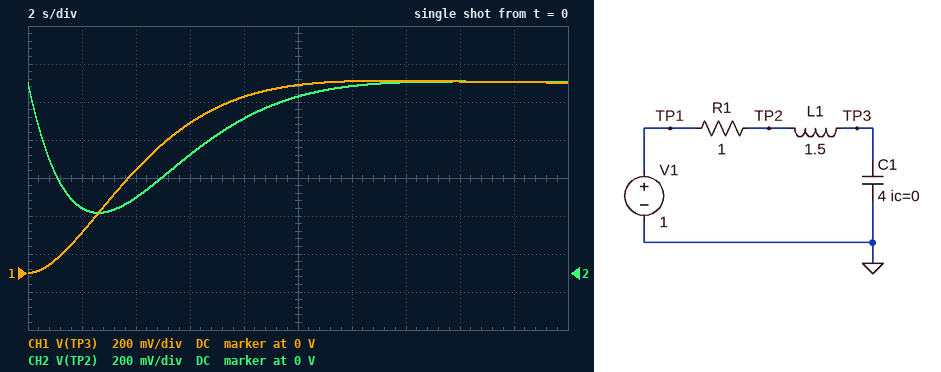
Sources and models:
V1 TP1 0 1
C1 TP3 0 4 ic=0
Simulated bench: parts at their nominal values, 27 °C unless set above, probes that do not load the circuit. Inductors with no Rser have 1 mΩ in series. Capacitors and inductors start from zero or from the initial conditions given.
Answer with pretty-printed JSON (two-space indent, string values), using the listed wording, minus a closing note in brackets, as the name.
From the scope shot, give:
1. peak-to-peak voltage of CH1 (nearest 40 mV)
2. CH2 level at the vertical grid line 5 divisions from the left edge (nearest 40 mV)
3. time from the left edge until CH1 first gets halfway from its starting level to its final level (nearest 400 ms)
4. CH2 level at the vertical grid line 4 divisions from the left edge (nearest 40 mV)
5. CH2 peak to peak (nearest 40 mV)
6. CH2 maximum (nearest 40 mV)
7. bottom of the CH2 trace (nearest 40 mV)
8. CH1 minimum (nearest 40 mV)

{
  "peak-to-peak voltage of CH1": "1.00 V",
  "CH2 level at the vertical grid line 5 divisions from the left edge": "920 mV",
  "time from the left edge until CH1 first gets halfway from its starting level to its final level": "3.6 s",
  "CH2 level at the vertical grid line 4 divisions from the left edge": "800 mV",
  "CH2 peak to peak": "680 mV",
  "CH2 maximum": "1.00 V",
  "bottom of the CH2 trace": "320 mV",
  "CH1 minimum": "0 V"
}
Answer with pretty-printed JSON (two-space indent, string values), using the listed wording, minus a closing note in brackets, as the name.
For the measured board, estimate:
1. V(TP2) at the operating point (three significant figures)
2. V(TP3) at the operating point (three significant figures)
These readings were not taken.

{
  "V(TP2) at the operating point": "1.00 V",
  "V(TP3) at the operating point": "1.00 V"
}
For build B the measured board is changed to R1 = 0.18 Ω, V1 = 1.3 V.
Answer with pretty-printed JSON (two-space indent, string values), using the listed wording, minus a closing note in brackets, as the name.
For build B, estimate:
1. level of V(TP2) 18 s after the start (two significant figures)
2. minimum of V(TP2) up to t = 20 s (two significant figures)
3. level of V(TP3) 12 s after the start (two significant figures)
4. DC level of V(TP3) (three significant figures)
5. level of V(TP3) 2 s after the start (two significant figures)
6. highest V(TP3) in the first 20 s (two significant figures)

{
  "level of V(TP2) 18 s after the start": "1.2 V",
  "minimum of V(TP2) up to t = 20 s": "990 mV",
  "level of V(TP3) 12 s after the start": "1.3 V",
  "DC level of V(TP3)": "1.30 V",
  "level of V(TP3) 2 s after the start": "380 mV",
  "highest V(TP3) in the first 20 s": "2.1 V"
}
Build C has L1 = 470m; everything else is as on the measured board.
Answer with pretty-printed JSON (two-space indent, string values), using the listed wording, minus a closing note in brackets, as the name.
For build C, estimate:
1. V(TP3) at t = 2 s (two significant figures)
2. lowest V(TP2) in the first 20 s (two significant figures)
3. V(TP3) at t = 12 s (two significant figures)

{
  "V(TP3) at t = 2 s": "340 mV",
  "lowest V(TP2) in the first 20 s": "180 mV",
  "V(TP3) at t = 12 s": "960 mV"
}
